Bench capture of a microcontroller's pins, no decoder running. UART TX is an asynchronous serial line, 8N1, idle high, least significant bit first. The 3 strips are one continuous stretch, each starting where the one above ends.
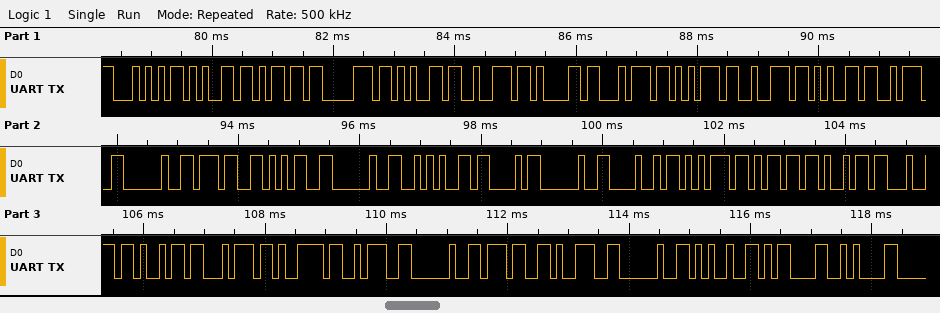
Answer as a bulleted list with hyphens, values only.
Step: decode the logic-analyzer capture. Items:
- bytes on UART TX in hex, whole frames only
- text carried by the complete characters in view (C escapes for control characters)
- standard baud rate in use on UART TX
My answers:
- 54 65 6D 70 65 72 61 74 75 72 65 3A 20 37 35 20 2A 43 20 48 75 6D 69 64 69 74 79 3A 20 37 39 20 25 0D 0A
- "Temperature: 75 *C Humidity: 79 %\r\n"
- 9600 baud
